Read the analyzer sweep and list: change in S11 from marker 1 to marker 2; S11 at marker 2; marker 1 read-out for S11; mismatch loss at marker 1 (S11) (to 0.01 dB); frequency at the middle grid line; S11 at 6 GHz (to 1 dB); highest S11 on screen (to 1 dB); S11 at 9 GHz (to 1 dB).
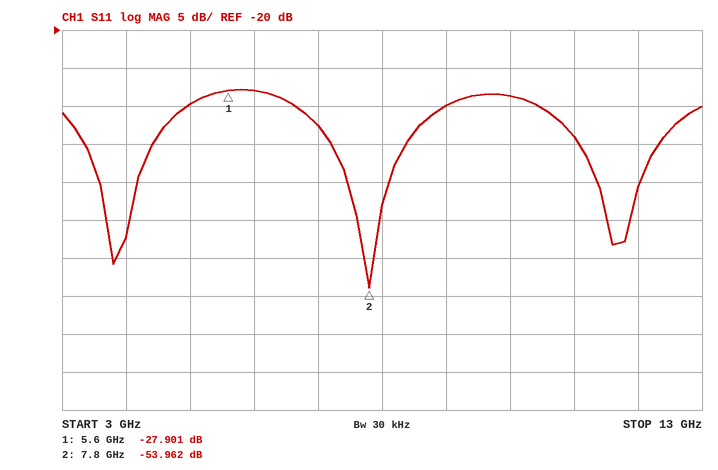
-26.061 dB
-53.962 dB
-27.901 dB
0.01 dB
8 GHz
-28 dB
-28 dB
-30 dB
